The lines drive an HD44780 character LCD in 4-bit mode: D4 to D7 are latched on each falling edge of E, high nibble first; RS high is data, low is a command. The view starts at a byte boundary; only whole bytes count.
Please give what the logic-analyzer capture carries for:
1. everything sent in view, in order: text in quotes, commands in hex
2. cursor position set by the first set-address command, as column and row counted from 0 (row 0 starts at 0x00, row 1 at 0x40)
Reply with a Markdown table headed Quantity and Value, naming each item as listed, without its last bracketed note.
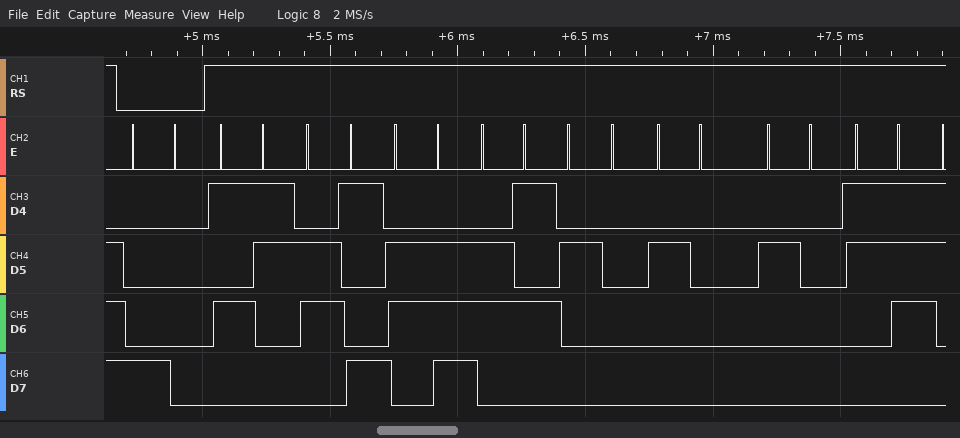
| Quantity | Value |
|---|---|
| everything sent in view, in order: text in quotes, commands in hex | 0x80 "Sine   7" |
| cursor position set by the first set-address command, as column and row counted from 0 | column 0, row 0 |
